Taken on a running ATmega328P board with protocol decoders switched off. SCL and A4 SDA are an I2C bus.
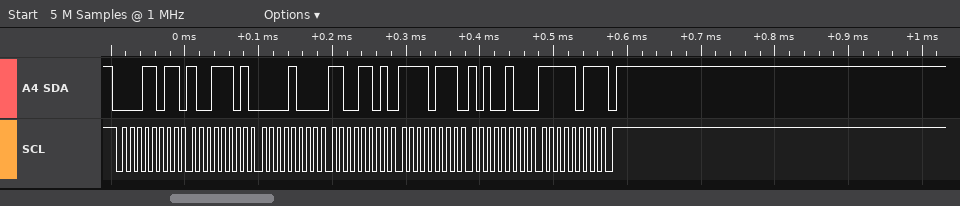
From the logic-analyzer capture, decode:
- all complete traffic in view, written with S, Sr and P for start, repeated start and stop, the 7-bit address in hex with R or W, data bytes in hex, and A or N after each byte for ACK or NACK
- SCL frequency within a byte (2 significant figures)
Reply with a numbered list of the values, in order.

1. S 0DR A 9D A 08 A CD A F7 A A4 A FB N P
2. 100 kHz
